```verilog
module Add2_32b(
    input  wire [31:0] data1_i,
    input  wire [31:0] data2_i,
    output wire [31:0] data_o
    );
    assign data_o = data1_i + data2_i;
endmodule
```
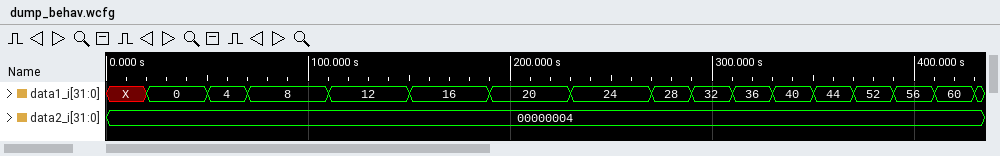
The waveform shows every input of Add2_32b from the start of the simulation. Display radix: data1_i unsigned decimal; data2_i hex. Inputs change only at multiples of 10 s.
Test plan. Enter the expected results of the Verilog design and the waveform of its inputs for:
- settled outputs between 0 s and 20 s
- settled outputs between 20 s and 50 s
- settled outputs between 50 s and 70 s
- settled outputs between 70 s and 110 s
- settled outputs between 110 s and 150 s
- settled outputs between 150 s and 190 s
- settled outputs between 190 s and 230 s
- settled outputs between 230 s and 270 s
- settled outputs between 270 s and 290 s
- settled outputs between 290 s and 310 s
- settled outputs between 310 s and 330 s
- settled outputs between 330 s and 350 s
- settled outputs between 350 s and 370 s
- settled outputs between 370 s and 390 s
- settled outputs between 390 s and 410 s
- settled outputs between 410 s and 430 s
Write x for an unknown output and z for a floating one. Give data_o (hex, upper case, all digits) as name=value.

data_o=x
data_o=00000004
data_o=00000008
data_o=0000000C
data_o=00000010
data_o=00000014
data_o=00000018
data_o=0000001C
data_o=00000020
data_o=00000024
data_o=00000028
data_o=0000002C
data_o=00000030
data_o=00000038
data_o=0000003C
data_o=00000040
